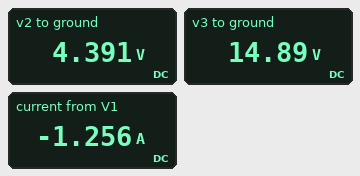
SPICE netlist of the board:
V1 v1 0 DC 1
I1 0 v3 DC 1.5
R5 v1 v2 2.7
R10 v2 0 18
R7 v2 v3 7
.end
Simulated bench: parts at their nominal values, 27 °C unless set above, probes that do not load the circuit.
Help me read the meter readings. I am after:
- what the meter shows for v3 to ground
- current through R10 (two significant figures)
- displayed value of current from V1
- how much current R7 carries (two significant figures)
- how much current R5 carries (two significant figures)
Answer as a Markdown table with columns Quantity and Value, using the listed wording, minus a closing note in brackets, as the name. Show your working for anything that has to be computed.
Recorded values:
| Quantity | Value |
|---|---|
| what the meter shows for v3 to ground | 14.89 V |
| current through R10 | (4.391 V) / 18 Ω = 240 mA |
| displayed value of current from V1 | -1.256 A |
| how much current R7 carries | (14.89 V - 4.391 V) / 7 Ω = 1.5 A |
| how much current R5 carries | (4.391 V - 1 V) / 2.7 Ω = 1.3 A |
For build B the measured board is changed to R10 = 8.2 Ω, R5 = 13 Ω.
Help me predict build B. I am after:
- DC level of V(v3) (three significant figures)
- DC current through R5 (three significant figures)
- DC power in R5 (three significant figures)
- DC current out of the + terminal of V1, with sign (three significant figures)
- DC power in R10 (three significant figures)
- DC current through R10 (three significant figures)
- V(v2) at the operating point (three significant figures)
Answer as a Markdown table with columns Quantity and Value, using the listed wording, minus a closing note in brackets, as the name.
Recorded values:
| Quantity | Value |
|---|---|
| DC level of V(v3) | 18.4 V |
| DC current through R5 | 533 mA |
| DC power in R5 | 3.69 W |
| DC current out of the + terminal of V1, with sign | -533 mA |
| DC power in R10 | 7.67 W |
| DC current through R10 | 967 mA |
| V(v2) at the operating point | 7.93 V |
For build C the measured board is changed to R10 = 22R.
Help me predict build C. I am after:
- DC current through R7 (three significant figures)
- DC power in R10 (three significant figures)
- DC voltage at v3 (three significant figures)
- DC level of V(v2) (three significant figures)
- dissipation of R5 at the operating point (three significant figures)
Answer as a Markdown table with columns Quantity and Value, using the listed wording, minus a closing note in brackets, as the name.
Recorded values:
| Quantity | Value |
|---|---|
| DC current through R7 | 1.50 A |
| DC power in R10 | 920 mW |
| DC voltage at v3 | 15.0 V |
| DC level of V(v2) | 4.50 V |
| dissipation of R5 at the operating point | 4.53 W |
